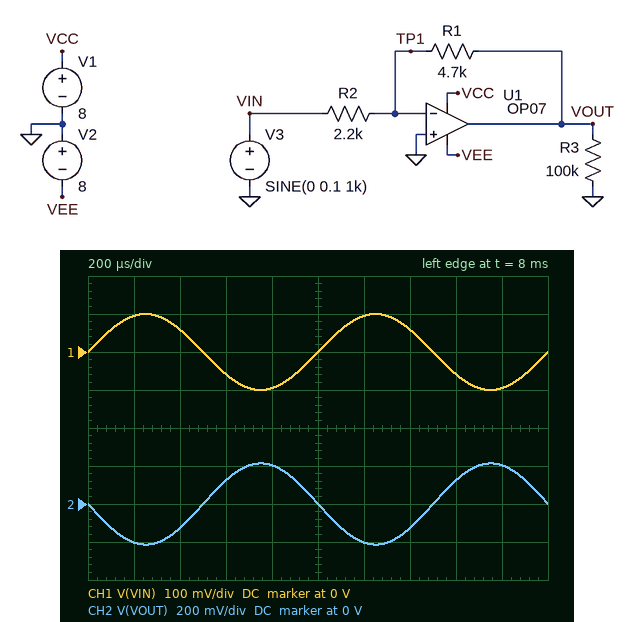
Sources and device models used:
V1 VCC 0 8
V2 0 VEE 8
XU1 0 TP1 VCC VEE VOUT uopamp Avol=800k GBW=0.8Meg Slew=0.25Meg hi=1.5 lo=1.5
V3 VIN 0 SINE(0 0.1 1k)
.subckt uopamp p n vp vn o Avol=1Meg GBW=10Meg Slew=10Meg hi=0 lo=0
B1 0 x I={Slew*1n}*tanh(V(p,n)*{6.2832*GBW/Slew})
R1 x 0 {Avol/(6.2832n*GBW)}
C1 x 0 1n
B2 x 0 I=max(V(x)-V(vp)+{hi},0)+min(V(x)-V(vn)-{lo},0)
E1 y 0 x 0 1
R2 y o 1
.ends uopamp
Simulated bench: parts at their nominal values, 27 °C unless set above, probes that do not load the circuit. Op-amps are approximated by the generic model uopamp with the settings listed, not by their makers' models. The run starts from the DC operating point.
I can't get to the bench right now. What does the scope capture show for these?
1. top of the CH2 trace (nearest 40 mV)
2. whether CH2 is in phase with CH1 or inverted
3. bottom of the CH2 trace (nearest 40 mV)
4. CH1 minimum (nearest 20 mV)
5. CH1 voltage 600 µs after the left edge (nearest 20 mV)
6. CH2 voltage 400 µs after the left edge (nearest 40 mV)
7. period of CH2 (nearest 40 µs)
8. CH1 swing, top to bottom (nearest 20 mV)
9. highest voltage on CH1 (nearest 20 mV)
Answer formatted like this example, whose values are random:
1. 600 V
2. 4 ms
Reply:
1. 200 mV
2. inverted
3. -200 mV
4. -100 mV
5. -60 mV
6. -120 mV
7. 1.00 ms
8. 200 mV
9. 100 mV
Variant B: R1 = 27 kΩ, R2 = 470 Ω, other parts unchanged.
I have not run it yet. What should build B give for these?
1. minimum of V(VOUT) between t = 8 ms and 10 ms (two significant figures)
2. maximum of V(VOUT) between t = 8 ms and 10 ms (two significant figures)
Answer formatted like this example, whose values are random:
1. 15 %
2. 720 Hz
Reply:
1. -5.7 V
2. 5.7 V
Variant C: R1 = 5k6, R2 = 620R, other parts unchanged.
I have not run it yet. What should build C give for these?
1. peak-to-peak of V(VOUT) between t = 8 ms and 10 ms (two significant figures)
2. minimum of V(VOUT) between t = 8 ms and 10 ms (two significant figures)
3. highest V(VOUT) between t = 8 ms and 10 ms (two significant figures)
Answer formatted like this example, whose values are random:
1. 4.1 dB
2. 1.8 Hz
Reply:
1. 1.8 V
2. -900 mV
3. 900 mV
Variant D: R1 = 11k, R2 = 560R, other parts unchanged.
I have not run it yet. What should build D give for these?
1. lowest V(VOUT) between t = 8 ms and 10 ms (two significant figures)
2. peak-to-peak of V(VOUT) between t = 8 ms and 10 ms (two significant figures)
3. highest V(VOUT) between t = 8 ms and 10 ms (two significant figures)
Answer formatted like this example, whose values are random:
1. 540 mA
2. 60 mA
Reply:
1. -2.0 V
2. 3.9 V
3. 2.0 V
